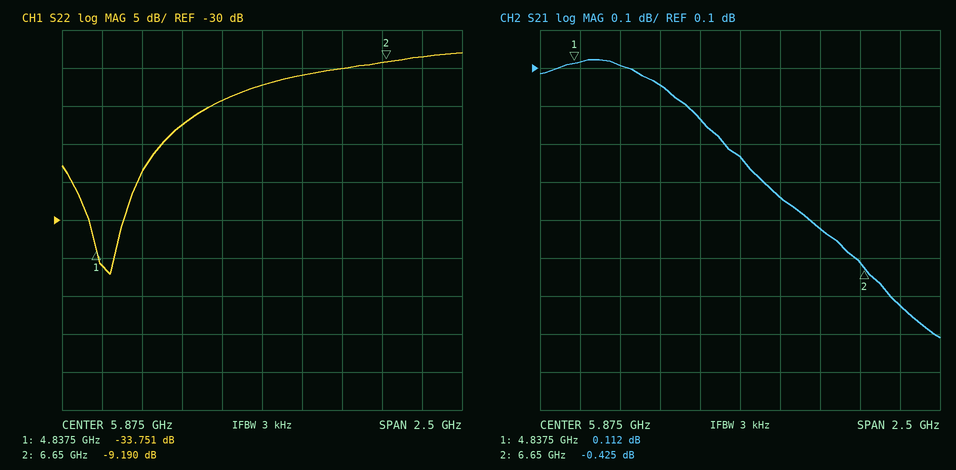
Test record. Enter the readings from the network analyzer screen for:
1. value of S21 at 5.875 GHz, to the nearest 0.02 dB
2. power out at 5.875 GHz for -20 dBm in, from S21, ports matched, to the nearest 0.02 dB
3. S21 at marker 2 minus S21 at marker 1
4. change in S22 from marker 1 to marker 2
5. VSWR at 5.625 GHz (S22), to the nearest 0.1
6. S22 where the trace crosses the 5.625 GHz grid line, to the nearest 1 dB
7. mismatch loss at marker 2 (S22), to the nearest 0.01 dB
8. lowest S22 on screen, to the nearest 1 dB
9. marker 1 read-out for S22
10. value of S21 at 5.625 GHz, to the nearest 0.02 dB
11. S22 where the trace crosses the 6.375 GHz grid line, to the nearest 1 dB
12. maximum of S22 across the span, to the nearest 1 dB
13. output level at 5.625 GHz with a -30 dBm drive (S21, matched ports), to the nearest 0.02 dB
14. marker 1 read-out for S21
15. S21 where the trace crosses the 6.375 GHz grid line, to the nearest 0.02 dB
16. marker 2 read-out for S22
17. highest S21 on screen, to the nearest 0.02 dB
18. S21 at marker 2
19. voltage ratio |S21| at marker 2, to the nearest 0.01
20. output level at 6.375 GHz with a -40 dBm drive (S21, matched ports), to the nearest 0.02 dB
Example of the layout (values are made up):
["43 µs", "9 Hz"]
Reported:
["-0.14 dB", "-20.14 dBm", "-0.537 dB", "24.561 dB", "1.5", "-14 dB", "0.56 dB", "-37 dB", "-33.751 dB", "-0.04 dB", "-10 dB", "-8 dB", "-30.04 dBm", "0.112 dB", "-0.32 dB", "-9.190 dB", "0.12 dB", "-0.425 dB", "0.95", "-40.32 dBm"]
